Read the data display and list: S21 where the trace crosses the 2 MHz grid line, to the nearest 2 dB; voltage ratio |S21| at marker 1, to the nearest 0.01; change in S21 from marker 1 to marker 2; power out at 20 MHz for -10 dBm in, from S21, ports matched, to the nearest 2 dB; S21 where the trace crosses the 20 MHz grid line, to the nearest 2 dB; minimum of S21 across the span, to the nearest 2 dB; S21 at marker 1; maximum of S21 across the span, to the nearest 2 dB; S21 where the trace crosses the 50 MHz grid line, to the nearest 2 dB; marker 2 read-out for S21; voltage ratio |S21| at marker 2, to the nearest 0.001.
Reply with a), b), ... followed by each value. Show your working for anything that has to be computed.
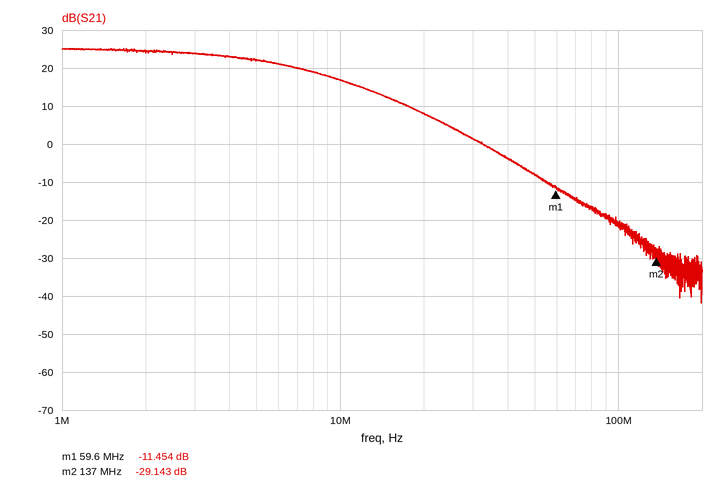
a) 24 dB
b) 10^(-11.454/20) ≈ 0.27
c) -29.143 − (-11.454) = -17.689 dB
d) -10 dBm + (8 dB) = -2 dBm
e) 8 dB
f) -42 dB
g) -11.454 dB
h) 26 dB
i) -8 dB
j) -29.143 dB
k) 10^(-29.143/20) ≈ 0.035
